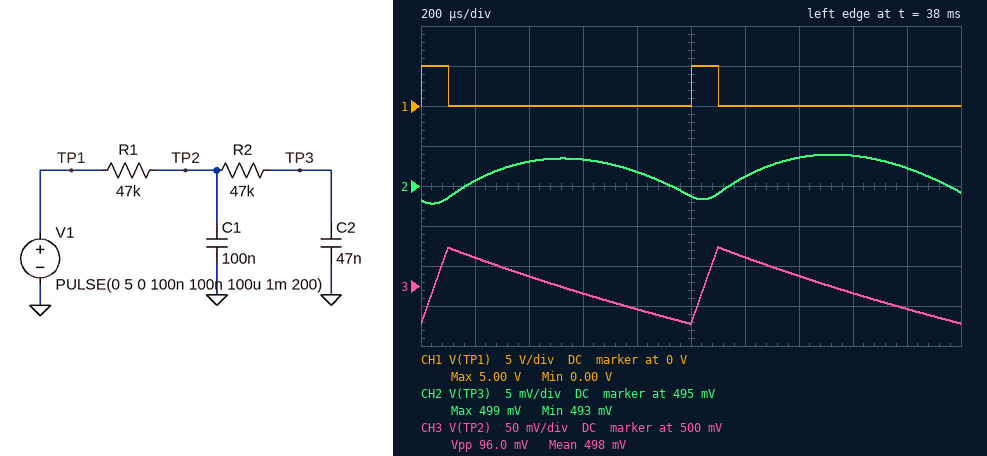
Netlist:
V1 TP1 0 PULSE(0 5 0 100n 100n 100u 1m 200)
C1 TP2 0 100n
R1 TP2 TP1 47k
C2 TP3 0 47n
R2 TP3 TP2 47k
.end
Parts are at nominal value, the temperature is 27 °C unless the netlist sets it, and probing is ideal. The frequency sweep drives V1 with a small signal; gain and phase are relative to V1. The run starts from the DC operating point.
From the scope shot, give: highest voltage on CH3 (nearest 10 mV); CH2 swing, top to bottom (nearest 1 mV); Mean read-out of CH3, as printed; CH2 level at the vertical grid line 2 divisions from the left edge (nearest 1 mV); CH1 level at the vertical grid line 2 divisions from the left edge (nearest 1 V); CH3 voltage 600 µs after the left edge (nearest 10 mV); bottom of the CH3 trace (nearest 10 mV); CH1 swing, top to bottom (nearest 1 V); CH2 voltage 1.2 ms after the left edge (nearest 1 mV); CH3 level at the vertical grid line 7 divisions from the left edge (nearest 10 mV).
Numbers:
550 mV
6 mV
498 mV
498 mV
0 V
490 mV
450 mV
5 V
496 mV
510 mV
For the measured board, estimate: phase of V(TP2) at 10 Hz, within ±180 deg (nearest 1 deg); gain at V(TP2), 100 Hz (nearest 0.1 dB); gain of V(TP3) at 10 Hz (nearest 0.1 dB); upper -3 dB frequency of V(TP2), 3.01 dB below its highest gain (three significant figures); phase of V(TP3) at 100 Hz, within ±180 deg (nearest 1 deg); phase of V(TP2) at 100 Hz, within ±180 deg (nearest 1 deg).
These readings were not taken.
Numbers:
-23 deg
-11.6 dB
-1.0 dB
21.5 Hz
-118 deg
-64 deg
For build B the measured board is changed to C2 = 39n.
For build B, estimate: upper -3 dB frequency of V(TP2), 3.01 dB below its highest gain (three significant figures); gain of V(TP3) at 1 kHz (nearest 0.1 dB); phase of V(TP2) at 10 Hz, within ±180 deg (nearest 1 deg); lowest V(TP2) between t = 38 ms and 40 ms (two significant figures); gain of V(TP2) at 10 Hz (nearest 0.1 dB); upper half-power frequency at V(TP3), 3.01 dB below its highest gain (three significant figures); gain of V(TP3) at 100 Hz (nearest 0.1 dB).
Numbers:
23.1 Hz
-50.7 dB
-22 deg
450 mV
-0.8 dB
21.6 Hz
-15.2 dB
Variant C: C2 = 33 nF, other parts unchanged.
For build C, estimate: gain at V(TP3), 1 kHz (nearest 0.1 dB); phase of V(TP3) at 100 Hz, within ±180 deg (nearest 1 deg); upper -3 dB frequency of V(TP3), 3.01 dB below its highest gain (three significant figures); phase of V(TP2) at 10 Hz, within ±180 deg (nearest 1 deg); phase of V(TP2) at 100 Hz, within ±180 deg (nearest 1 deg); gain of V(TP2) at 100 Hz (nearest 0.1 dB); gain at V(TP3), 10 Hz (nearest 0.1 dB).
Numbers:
-49.3 dB
-111 deg
23.1 Hz
-21 deg
-67 deg
-11.5 dB
-0.7 dB
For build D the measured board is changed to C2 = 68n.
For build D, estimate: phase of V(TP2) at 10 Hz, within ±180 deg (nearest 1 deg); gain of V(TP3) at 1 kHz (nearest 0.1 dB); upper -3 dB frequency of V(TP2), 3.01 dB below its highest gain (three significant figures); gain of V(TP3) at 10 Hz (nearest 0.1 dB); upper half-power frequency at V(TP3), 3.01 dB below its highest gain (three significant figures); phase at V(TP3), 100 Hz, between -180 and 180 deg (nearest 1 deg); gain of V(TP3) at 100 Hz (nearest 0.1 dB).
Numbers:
-25 deg
-55.5 dB
18.3 Hz
-1.4 dB
16.3 Hz
-125 deg
-18.6 dB
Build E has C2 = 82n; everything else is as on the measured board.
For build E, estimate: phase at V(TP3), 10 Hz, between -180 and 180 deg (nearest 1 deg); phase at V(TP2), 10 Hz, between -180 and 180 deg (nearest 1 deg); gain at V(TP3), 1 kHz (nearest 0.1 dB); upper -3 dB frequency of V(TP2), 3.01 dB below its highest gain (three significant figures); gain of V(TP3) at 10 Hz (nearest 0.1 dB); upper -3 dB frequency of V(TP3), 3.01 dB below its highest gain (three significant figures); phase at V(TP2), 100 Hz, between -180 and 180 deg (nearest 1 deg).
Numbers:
-40 deg
-26 deg
-57.1 dB
16.6 Hz
-1.7 dB
14.5 Hz
-61 deg
